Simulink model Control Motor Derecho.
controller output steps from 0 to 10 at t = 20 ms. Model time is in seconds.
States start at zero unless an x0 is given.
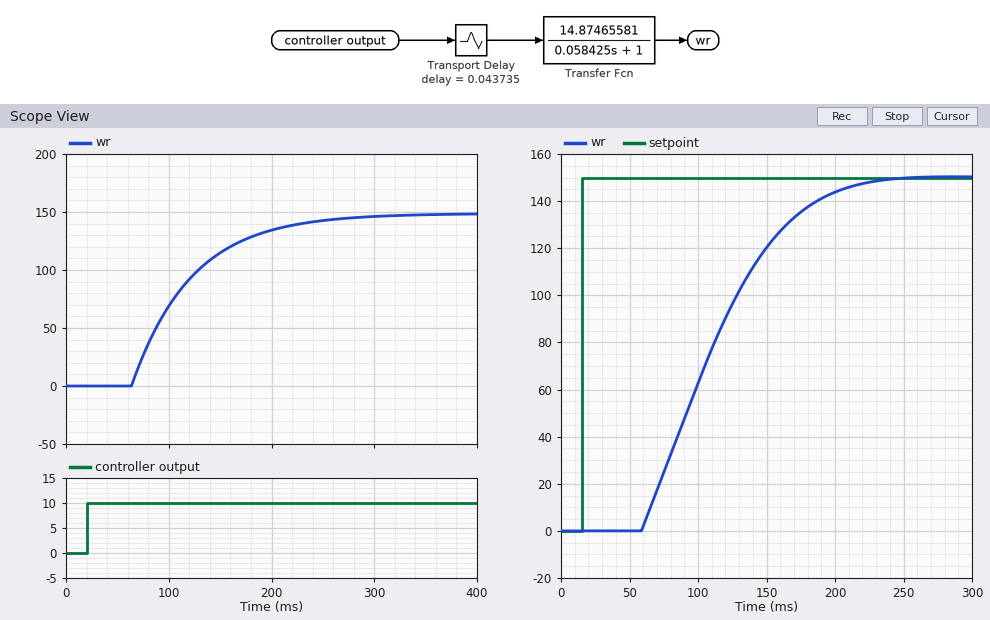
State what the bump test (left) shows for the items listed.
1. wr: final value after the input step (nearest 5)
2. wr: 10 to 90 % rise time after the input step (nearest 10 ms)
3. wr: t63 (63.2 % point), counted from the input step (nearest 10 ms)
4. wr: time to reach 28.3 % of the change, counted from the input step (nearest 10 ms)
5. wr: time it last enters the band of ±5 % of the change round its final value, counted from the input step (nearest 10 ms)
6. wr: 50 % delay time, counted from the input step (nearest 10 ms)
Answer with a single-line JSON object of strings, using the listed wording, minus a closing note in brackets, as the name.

{"wr: final value after the input step": "150", "wr: 10 to 90 % rise time after the input step": "130 ms", "wr: t63 (63.2 % point), counted from the input step": "100 ms", "wr: time to reach 28.3 % of the change, counted from the input step": "60 ms", "wr: time it last enters the band of ±5 % of the change round its final value, counted from the input step": "220 ms", "wr: 50 % delay time, counted from the input step": "80 ms"}
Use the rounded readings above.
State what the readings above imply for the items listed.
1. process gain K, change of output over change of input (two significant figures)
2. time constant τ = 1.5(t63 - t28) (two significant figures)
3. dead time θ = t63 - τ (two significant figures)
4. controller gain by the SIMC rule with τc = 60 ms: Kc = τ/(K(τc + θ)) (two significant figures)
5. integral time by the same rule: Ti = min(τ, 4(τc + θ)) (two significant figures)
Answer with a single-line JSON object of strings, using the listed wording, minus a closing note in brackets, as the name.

{"process gain K, change of output over change of input": "15", "time constant τ = 1.5(t63 - t28)": "60 ms", "dead time θ = t63 - τ": "40 ms", "controller gain by the SIMC rule with τc = 60 ms: Kc = τ/(K(τc + θ))": "0.040", "integral time by the same rule: Ti = min(τ, 4(τc + θ))": "60 ms"}
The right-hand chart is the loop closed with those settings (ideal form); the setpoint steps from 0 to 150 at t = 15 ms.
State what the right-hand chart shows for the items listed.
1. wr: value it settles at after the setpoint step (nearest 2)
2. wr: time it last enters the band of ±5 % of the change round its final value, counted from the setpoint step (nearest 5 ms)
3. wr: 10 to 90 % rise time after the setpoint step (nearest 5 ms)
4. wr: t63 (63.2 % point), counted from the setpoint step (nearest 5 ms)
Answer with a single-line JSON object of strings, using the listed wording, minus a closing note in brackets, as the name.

{"wr: value it settles at after the setpoint step": "150", "wr: time it last enters the band of ±5 % of the change round its final value, counted from the setpoint step": "180 ms", "wr: 10 to 90 % rise time after the setpoint step": "105 ms", "wr: t63 (63.2 % point), counted from the setpoint step": "110 ms"}
